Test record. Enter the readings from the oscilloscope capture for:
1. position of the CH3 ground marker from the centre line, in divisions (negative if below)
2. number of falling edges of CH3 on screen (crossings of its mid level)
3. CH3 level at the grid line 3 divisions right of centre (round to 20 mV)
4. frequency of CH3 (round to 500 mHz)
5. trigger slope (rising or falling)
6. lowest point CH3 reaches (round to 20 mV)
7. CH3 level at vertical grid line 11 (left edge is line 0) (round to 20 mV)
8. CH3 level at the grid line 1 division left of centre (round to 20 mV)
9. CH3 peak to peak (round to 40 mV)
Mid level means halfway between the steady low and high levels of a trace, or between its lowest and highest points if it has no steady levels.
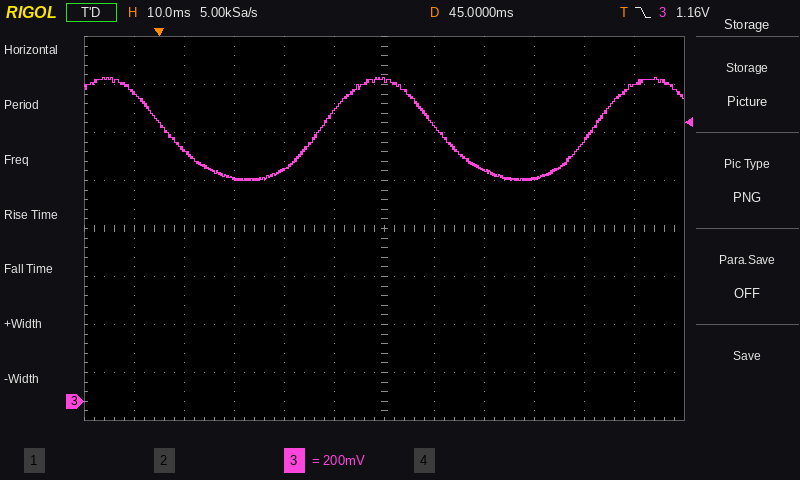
-3.6 div
2
920 mV
18.5 Hz
falling
920 mV
1.32 V
1.22 V
440 mV
